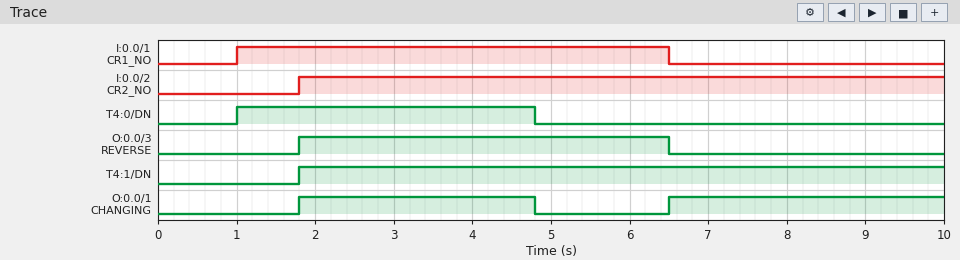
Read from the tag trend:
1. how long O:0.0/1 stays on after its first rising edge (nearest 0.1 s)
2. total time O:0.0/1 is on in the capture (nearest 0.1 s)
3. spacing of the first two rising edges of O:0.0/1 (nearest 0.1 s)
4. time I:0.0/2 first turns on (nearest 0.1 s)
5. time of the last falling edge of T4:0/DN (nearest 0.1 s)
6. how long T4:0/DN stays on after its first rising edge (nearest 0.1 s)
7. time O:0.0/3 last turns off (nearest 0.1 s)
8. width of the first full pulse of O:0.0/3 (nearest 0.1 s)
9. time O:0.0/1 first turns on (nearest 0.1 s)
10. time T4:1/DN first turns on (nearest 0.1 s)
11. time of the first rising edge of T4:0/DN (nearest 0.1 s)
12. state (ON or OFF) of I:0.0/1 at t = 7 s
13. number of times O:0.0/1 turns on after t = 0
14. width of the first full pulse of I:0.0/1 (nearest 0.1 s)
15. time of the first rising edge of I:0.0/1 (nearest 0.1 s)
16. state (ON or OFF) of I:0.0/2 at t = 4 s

3.0 s
6.5 s
4.7 s
1.8 s
4.8 s
3.8 s
6.5 s
4.7 s
1.8 s
1.8 s
1.0 s
OFF
2
5.5 s
1.0 s
ON
